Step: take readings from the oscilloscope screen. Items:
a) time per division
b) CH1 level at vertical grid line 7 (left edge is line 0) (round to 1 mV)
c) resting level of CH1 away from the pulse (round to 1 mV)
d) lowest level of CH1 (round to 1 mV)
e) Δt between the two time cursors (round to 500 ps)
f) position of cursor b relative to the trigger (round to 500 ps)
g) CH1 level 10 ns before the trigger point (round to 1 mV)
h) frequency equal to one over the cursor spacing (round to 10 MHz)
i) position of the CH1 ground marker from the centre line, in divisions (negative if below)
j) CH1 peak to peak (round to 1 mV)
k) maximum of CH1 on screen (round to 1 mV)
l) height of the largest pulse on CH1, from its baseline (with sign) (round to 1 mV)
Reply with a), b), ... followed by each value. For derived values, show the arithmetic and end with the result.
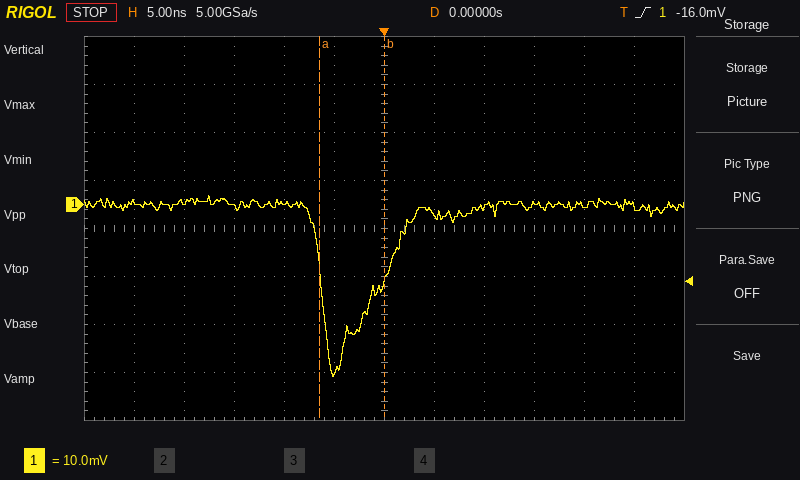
a) 5 ns
b) -2 mV
c) 0 mV
d) -36 mV
e) 6.5 ns
f) 0.0 ns
g) 0 mV
h) 1 / 6.5 ns ≈ 150 MHz
i) +0.5 div
j) 2 mV − (-36 mV) = 38 mV
k) 2 mV
l) -36 mV − (0 mV) = -36 mV
